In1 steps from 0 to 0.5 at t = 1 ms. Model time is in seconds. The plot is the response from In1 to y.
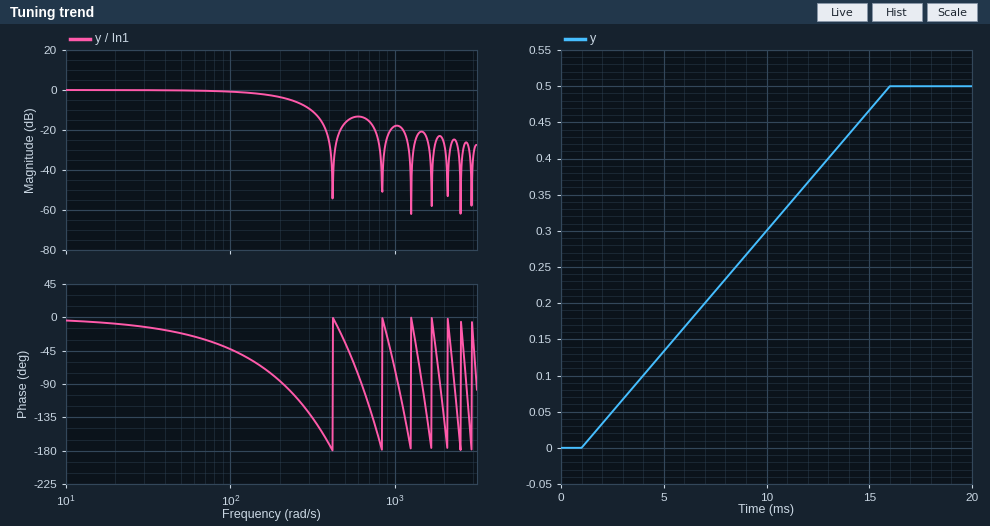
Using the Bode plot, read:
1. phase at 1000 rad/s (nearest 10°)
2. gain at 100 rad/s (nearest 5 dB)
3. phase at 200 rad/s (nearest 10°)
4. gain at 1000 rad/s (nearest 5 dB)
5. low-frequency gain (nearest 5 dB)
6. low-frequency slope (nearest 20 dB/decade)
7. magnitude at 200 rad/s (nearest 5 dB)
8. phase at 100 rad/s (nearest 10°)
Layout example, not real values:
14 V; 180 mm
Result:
-70°; 0 dB; -90°; -20 dB; 0 dB; 0 dB/decade; -5 dB; -40°
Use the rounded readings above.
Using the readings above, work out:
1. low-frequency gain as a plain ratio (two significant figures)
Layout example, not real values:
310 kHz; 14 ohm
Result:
1.0
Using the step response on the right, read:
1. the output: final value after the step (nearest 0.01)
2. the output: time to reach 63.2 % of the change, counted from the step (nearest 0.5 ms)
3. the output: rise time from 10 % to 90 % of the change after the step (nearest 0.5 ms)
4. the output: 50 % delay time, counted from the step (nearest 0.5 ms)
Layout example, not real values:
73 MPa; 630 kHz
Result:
0.50; 9.5 ms; 12.0 ms; 7.5 ms
